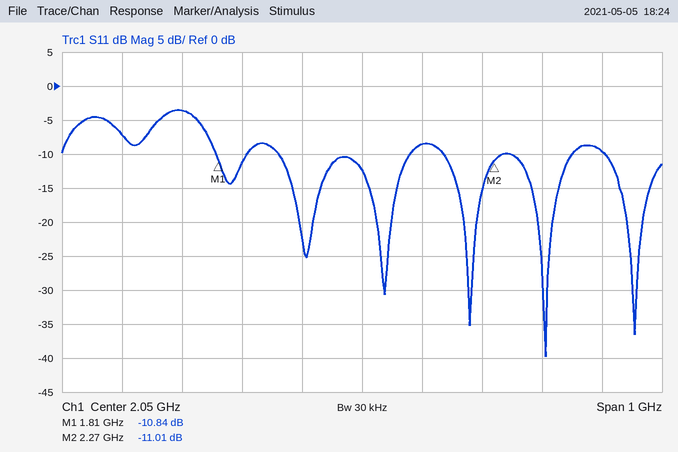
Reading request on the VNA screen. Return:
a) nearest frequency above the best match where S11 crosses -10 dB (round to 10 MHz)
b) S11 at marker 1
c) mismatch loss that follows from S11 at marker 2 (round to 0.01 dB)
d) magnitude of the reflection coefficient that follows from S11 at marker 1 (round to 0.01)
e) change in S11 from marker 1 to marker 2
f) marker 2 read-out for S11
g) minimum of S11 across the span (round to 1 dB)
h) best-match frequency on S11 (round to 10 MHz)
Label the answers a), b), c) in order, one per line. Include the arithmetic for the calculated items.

a) 2.40 GHz
b) -10.84 dB
c) −10 log10(1 − 10^(-11.01/10)) ≈ 0.36 dB
d) 10^(-10.84/20) ≈ 0.29
e) -11.01 − (-10.84) = -0.17 dB
f) -11.01 dB
g) -40 dB
h) 2.36 GHz
